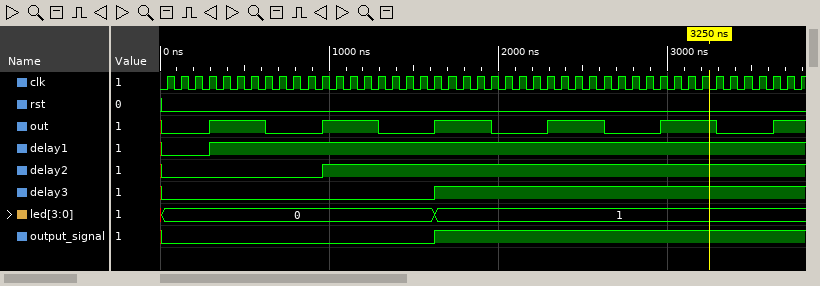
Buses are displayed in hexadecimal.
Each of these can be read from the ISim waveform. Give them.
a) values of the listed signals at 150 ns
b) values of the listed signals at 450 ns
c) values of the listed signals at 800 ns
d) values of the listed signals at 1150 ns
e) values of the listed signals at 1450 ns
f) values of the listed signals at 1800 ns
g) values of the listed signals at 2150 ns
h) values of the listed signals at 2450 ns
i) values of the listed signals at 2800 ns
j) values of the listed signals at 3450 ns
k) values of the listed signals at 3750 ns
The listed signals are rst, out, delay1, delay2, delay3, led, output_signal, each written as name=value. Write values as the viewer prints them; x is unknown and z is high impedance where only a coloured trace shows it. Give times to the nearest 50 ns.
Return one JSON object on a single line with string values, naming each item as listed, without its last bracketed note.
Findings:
{"values of the listed signals at 150 ns": "rst=0, out=0, delay1=0, delay2=0, delay3=0, led=0, output_signal=0", "values of the listed signals at 450 ns": "rst=0, out=1, delay1=1, delay2=0, delay3=0, led=0, output_signal=0", "values of the listed signals at 800 ns": "rst=0, out=0, delay1=1, delay2=0, delay3=0, led=0, output_signal=0", "values of the listed signals at 1150 ns": "rst=0, out=1, delay1=1, delay2=1, delay3=0, led=0, output_signal=0", "values of the listed signals at 1450 ns": "rst=0, out=0, delay1=1, delay2=1, delay3=0, led=0, output_signal=0", "values of the listed signals at 1800 ns": "rst=0, out=1, delay1=1, delay2=1, delay3=1, led=1, output_signal=1", "values of the listed signals at 2150 ns": "rst=0, out=0, delay1=1, delay2=1, delay3=1, led=1, output_signal=1", "values of the listed signals at 2450 ns": "rst=0, out=1, delay1=1, delay2=1, delay3=1, led=1, output_signal=1", "values of the listed signals at 2800 ns": "rst=0, out=0, delay1=1, delay2=1, delay3=1, led=1, output_signal=1", "values of the listed signals at 3450 ns": "rst=0, out=0, delay1=1, delay2=1, delay3=1, led=1, output_signal=1", "values of the listed signals at 3750 ns": "rst=0, out=1, delay1=1, delay2=1, delay3=1, led=1, output_signal=1"}
